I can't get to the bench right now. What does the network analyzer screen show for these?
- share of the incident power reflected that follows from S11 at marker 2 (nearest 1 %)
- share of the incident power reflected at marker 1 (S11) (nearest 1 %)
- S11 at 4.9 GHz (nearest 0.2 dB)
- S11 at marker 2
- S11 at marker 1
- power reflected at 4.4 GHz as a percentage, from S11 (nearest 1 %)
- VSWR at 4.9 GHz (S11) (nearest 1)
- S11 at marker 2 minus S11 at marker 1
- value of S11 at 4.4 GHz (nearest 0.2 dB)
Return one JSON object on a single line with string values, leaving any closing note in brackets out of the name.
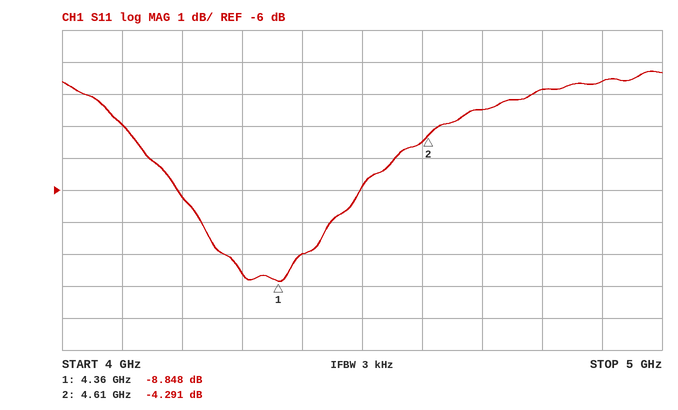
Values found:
{"share of the incident power reflected that follows from S11 at marker 2": "37 %", "share of the incident power reflected at marker 1 (S11)": "13 %", "S11 at 4.9 GHz": "-2.6 dB", "S11 at marker 2": "-4.291 dB", "S11 at marker 1": "-8.848 dB", "power reflected at 4.4 GHz as a percentage, from S11": "16 %", "VSWR at 4.9 GHz (S11)": "7", "S11 at marker 2 minus S11 at marker 1": "4.557 dB", "value of S11 at 4.4 GHz": "-8.0 dB"}
